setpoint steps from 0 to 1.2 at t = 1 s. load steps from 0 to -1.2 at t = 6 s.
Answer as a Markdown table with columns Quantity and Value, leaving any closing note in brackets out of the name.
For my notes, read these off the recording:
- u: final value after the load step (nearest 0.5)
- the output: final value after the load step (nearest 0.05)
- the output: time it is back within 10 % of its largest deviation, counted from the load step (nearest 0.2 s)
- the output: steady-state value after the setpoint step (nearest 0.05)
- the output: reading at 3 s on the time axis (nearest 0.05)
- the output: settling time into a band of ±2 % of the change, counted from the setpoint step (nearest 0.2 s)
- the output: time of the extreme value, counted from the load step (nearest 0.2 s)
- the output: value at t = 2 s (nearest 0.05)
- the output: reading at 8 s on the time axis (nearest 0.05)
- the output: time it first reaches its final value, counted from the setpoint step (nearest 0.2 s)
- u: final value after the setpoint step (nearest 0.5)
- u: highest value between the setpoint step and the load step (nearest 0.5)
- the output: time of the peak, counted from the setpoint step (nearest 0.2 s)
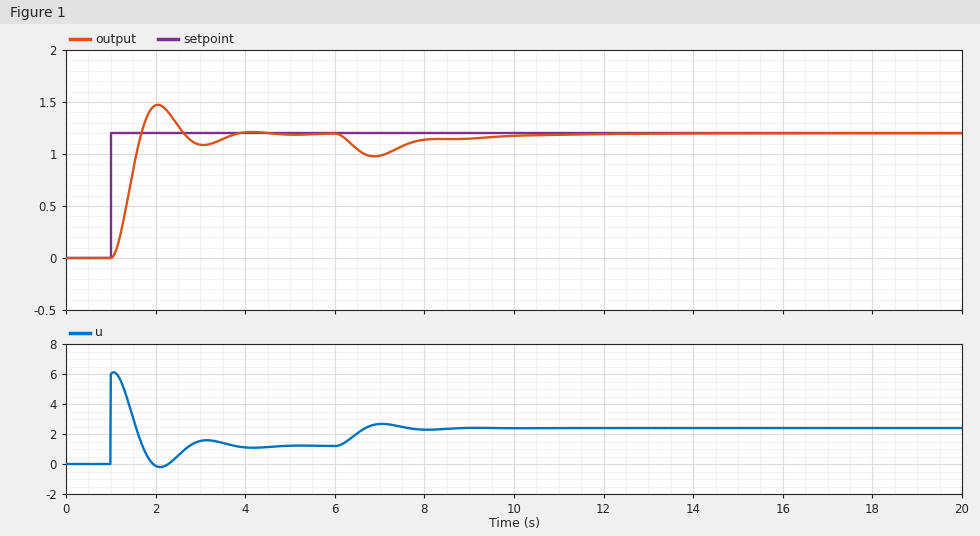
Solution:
| Quantity | Value |
|---|---|
| u: final value after the load step | 2.5 |
| the output: final value after the load step | 1.20 |
| the output: time it is back within 10 % of its largest deviation, counted from the load step | 4.2 s |
| the output: steady-state value after the setpoint step | 1.20 |
| the output: reading at 3 s on the time axis | 1.10 |
| the output: settling time into a band of ±2 % of the change, counted from the setpoint step | 2.6 s |
| the output: time of the extreme value, counted from the load step | 0.8 s |
| the output: value at t = 2 s | 1.45 |
| the output: reading at 8 s on the time axis | 1.15 |
| the output: time it first reaches its final value, counted from the setpoint step | 0.6 s |
| u: final value after the setpoint step | 1.0 |
| u: highest value between the setpoint step and the load step | 6.0 |
| the output: time of the peak, counted from the setpoint step | 1.0 s |
